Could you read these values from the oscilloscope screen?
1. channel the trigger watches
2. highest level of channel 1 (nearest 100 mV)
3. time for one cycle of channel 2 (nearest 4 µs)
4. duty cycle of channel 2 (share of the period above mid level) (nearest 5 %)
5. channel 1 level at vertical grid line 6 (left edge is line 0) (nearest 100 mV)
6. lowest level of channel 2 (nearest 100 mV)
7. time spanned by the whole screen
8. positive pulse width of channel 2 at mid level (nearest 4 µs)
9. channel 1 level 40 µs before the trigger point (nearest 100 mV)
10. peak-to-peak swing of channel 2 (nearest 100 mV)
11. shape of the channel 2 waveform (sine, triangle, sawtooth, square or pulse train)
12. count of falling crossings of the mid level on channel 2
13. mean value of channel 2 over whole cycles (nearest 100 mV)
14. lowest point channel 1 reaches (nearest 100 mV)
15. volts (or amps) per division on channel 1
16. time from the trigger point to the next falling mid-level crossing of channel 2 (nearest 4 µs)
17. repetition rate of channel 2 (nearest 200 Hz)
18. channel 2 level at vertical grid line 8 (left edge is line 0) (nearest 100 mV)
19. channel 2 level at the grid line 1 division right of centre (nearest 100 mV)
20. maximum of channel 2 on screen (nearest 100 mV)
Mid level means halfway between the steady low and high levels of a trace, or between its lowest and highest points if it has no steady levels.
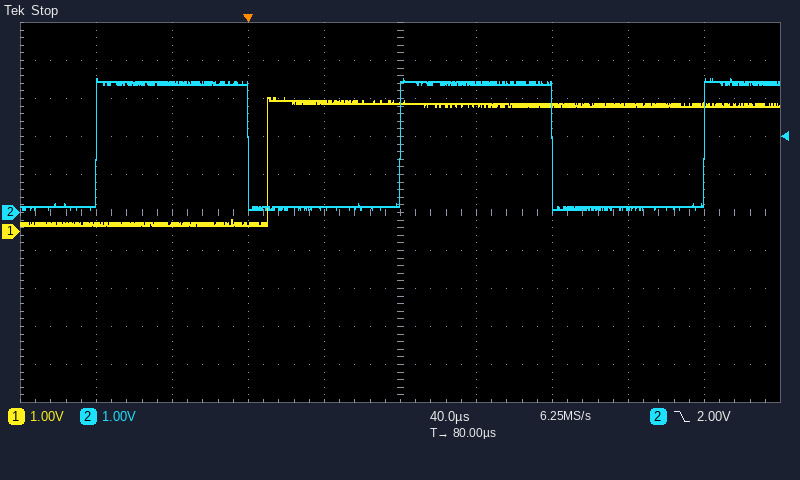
channel 2
3.5 V
160 µs
50 %
3.3 V
0.0 V
400 µs
80 µs
200 mV
3.5 V
square
2
1.8 V
200 mV
1 V
160 µs
6.2 kHz
100 mV
3.4 V
3.5 V
